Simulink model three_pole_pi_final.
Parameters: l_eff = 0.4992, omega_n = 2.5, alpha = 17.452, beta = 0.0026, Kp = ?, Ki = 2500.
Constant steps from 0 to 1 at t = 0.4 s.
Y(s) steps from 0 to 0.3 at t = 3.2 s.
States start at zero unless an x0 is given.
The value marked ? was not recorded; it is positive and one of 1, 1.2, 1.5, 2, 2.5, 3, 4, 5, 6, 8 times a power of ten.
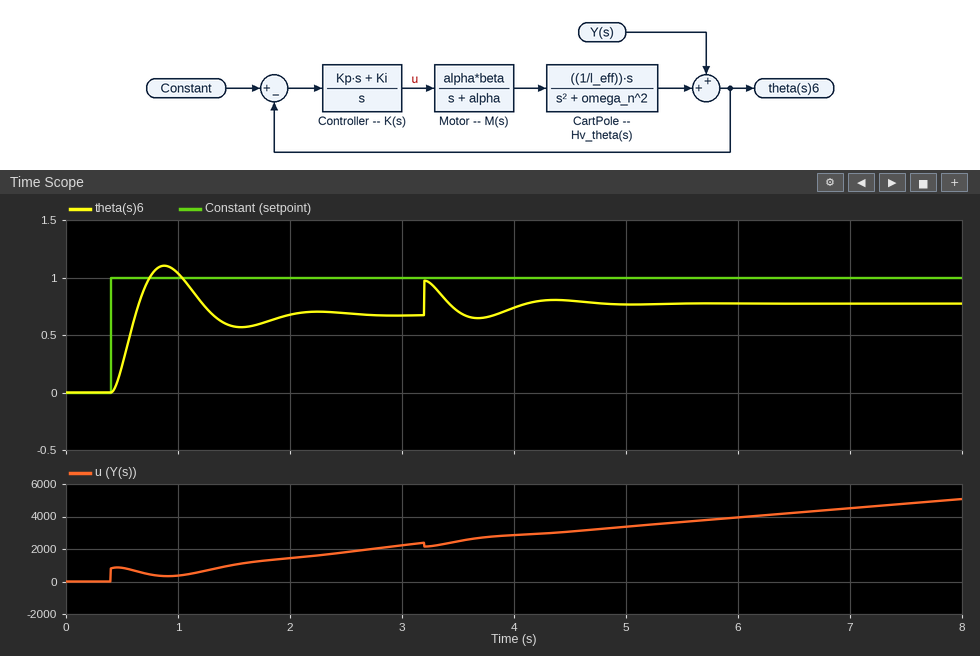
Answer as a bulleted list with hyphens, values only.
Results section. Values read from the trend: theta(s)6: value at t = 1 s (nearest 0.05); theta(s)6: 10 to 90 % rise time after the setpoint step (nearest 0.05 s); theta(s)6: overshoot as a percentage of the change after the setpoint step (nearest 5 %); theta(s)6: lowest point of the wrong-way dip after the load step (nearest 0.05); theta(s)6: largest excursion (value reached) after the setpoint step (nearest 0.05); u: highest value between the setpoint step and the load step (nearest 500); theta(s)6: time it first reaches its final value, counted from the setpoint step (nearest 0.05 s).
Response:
- 1.05
- 0.15 s
- 65 %
- 0.65
- 1.10
- 2500
- 0.20 s
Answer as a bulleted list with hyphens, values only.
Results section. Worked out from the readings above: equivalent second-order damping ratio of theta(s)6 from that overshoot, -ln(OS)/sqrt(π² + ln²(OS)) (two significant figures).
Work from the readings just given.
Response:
- 0.14
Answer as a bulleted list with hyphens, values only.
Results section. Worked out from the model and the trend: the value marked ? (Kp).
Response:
- 800
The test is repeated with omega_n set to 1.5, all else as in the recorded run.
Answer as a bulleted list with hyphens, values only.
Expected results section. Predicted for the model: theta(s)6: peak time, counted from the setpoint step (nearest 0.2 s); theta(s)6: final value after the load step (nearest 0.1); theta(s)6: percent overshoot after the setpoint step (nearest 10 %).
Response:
- 0.6 s
- 0.9
- 50 %
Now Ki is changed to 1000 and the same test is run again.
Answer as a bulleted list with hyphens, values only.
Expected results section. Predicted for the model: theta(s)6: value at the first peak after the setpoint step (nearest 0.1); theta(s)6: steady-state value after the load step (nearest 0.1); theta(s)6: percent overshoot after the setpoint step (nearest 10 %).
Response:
- 0.9
- 0.6
- 100 %
